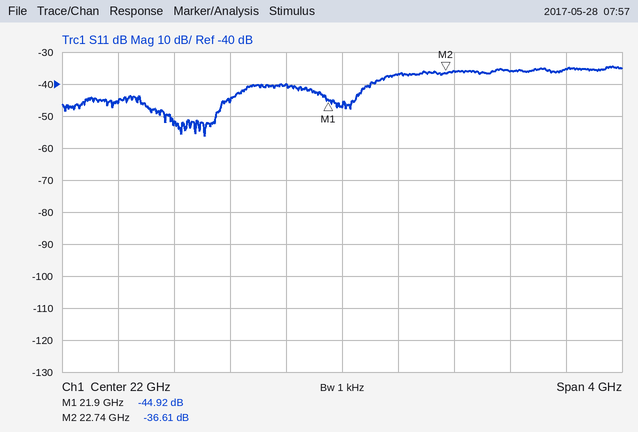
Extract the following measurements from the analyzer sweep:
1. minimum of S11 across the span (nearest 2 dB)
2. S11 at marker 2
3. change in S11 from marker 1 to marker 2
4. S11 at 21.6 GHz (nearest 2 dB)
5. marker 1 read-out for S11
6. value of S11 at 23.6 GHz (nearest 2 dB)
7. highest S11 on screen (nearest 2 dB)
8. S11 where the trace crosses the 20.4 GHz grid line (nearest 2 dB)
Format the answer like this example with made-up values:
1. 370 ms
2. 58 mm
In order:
1. -56 dB
2. -36.61 dB
3. 8.31 dB
4. -40 dB
5. -44.92 dB
6. -36 dB
7. -34 dB
8. -46 dB
